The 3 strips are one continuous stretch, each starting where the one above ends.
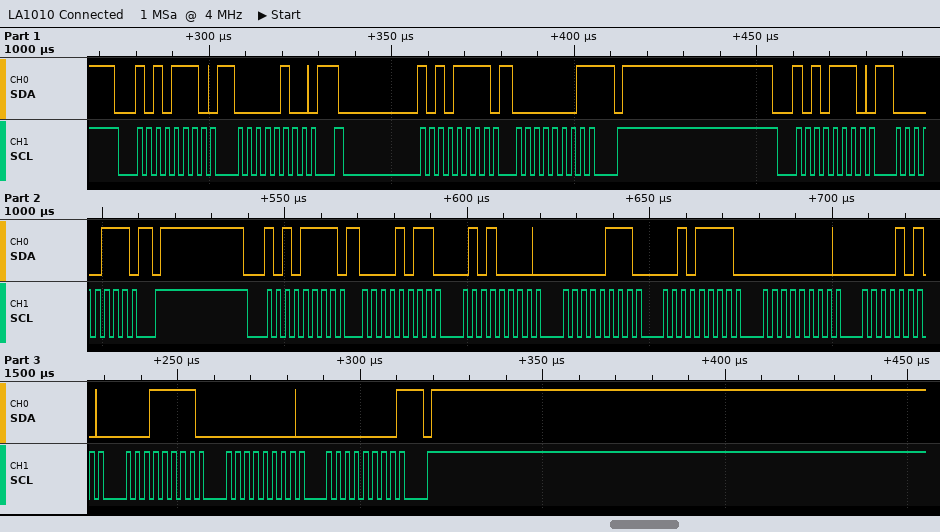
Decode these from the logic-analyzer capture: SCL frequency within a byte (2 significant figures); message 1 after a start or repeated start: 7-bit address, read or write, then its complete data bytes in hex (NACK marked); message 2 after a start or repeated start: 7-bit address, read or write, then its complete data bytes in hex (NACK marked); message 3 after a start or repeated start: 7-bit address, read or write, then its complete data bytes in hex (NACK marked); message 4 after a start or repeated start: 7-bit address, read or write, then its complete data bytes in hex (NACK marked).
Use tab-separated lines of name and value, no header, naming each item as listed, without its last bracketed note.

SCL frequency within a byte	400 kHz
message 1 after a start or repeated start: 7-bit address, read or write, then its complete data bytes in hex	0x57 write: 04
message 2 after a start or repeated start: 7-bit address, read or write, then its complete data bytes in hex	0x57 read: 01 NACK
message 3 after a start or repeated start: 7-bit address, read or write, then its complete data bytes in hex	0x57 write: 07
message 4 after a start or repeated start: 7-bit address, read or write, then its complete data bytes in hex	0x57 read: 0B 50 07 2F 00 0A 1F 00 00 NACK
